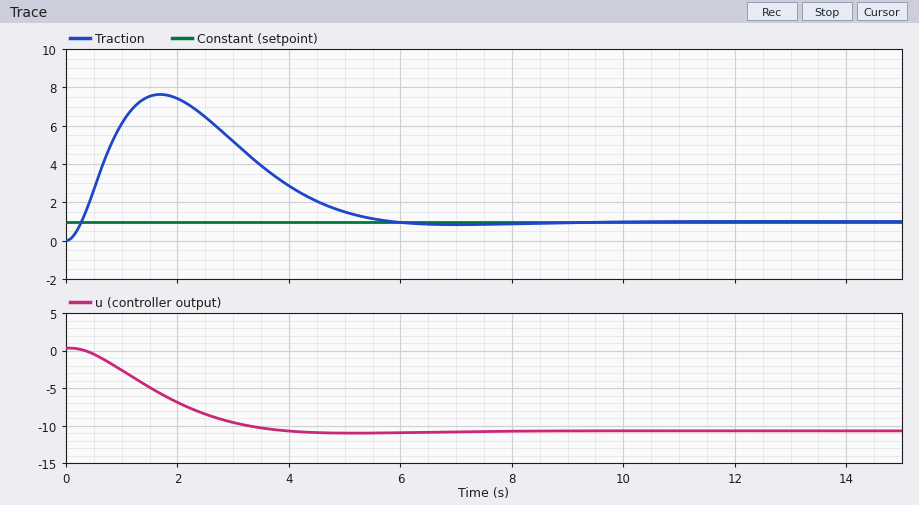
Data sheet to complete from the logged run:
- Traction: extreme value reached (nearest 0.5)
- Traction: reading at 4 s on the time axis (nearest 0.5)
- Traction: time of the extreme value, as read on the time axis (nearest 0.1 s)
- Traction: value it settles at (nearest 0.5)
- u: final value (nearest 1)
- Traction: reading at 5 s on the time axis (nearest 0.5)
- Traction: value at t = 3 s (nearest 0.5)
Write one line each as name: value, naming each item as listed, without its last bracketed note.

Traction: extreme value reached: 7.5
Traction: reading at 4 s on the time axis: 3.0
Traction: time of the extreme value, as read on the time axis: 1.7 s
Traction: value it settles at: 1.0
u: final value: -11
Traction: reading at 5 s on the time axis: 1.5
Traction: value at t = 3 s: 5.0
